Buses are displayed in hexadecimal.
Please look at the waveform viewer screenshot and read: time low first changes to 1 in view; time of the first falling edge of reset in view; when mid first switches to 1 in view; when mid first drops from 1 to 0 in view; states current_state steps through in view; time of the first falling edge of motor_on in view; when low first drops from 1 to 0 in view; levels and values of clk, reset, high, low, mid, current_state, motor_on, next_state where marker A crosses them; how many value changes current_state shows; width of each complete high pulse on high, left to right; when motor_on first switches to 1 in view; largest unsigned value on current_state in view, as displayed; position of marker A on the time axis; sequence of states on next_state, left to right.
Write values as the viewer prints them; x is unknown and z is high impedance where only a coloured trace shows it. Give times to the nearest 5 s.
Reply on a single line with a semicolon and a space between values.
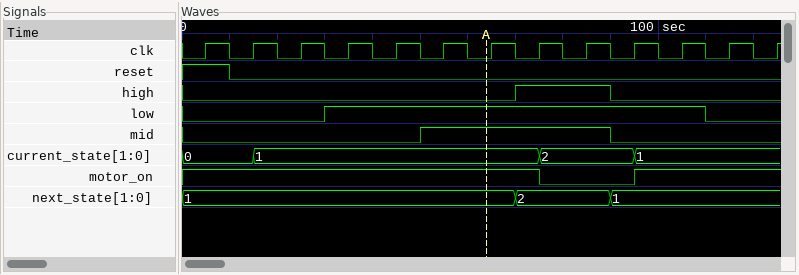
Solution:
30 s; 10 s; 50 s; 90 s; 0, 1, 2, 1; 75 s; 110 s; clk=0, reset=0, high=0, low=1, mid=1, current_state=1, motor_on=1, next_state=1; 3; 20 s; 95 s; 2; 65 s; 1, 2, 1
